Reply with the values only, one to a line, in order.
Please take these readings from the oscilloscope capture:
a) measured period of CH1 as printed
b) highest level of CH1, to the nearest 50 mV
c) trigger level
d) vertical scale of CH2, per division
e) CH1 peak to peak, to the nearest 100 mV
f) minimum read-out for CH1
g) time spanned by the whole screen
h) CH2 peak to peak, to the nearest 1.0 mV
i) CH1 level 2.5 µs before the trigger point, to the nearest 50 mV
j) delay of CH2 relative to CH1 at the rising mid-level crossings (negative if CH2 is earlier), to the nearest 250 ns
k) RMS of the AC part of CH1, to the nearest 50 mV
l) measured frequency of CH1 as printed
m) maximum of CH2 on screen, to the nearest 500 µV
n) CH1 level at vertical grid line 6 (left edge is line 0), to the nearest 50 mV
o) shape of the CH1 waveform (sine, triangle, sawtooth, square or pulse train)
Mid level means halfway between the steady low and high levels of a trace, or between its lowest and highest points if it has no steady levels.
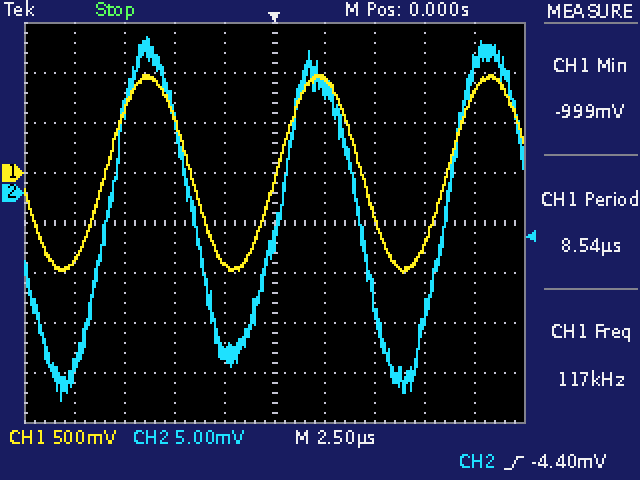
8.54 µs
1.00 V
-4.40 mV
5 mV
2.00 V
-999 mV
25 µs
36.0 mV
-900 mV
0.00 µs
700 mV
117 kHz
15.5 mV
950 mV
sine
